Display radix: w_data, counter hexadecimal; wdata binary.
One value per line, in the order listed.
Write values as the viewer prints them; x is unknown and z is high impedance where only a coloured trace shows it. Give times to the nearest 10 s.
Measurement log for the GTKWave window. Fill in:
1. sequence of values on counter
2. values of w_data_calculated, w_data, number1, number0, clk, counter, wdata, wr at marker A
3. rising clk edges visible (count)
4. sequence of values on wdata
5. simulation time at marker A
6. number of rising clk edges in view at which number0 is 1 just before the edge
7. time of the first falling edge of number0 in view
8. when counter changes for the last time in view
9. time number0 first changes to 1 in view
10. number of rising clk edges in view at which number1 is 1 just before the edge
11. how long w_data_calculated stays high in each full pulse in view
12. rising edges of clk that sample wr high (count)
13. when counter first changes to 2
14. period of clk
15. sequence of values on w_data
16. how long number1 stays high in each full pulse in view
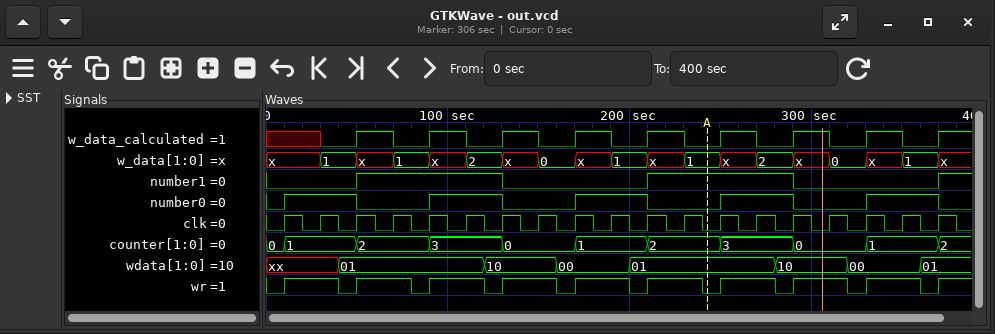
0, 1, 2, 3, 0, 1, 2, 3, 0, 1, 2
w_data_calculated=0, w_data=1, number1=1, number0=0, clk=0, counter=2, wdata=01, wr=0
19
xx, 01, 10, 00, 01, 10, 00, 01
240 s
10
50 s
370 s
10 s
8
20 s, 20 s, 20 s, 20 s, 20 s, 20 s, 20 s, 20 s
9
50 s
20 s
x, 1, x, 1, x, 2, x, 0, x, 1, x, 1, x, 2, x, 0, x, 1, x
80 s, 80 s
